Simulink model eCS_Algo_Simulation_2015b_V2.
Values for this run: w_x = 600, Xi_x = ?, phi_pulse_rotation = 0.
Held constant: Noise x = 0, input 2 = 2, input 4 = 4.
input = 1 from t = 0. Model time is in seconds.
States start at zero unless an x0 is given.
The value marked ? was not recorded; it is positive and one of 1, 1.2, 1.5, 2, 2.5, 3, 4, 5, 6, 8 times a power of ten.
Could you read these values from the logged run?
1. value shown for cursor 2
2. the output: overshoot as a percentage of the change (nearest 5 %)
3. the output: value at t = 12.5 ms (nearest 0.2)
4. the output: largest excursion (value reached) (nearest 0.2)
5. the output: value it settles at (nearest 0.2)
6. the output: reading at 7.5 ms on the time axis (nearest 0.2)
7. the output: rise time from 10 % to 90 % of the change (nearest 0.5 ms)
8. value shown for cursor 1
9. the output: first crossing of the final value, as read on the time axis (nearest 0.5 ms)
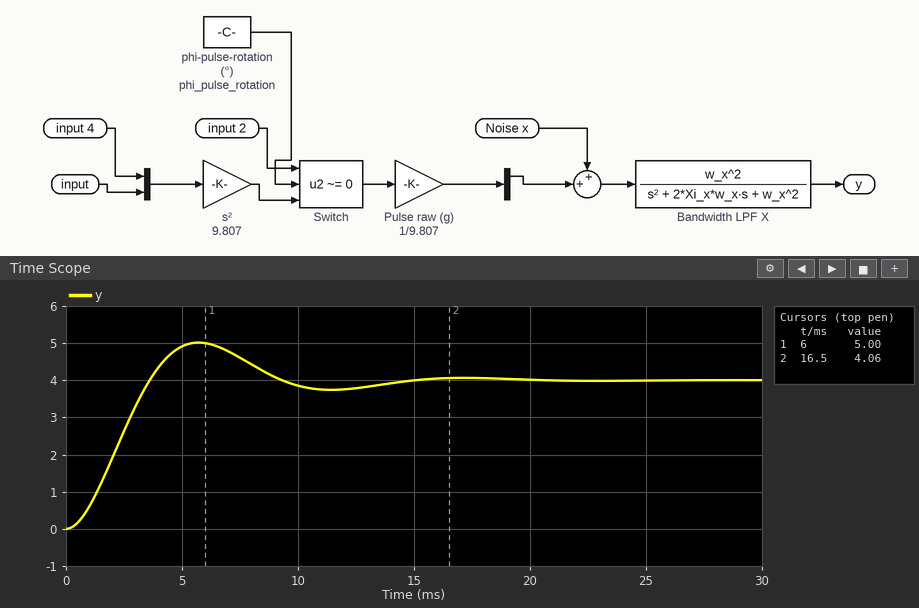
4.06
25 %
3.8
5.0
4.0
4.6
2.5 ms
5.00
3.5 ms
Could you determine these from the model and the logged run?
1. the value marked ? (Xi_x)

0.4
